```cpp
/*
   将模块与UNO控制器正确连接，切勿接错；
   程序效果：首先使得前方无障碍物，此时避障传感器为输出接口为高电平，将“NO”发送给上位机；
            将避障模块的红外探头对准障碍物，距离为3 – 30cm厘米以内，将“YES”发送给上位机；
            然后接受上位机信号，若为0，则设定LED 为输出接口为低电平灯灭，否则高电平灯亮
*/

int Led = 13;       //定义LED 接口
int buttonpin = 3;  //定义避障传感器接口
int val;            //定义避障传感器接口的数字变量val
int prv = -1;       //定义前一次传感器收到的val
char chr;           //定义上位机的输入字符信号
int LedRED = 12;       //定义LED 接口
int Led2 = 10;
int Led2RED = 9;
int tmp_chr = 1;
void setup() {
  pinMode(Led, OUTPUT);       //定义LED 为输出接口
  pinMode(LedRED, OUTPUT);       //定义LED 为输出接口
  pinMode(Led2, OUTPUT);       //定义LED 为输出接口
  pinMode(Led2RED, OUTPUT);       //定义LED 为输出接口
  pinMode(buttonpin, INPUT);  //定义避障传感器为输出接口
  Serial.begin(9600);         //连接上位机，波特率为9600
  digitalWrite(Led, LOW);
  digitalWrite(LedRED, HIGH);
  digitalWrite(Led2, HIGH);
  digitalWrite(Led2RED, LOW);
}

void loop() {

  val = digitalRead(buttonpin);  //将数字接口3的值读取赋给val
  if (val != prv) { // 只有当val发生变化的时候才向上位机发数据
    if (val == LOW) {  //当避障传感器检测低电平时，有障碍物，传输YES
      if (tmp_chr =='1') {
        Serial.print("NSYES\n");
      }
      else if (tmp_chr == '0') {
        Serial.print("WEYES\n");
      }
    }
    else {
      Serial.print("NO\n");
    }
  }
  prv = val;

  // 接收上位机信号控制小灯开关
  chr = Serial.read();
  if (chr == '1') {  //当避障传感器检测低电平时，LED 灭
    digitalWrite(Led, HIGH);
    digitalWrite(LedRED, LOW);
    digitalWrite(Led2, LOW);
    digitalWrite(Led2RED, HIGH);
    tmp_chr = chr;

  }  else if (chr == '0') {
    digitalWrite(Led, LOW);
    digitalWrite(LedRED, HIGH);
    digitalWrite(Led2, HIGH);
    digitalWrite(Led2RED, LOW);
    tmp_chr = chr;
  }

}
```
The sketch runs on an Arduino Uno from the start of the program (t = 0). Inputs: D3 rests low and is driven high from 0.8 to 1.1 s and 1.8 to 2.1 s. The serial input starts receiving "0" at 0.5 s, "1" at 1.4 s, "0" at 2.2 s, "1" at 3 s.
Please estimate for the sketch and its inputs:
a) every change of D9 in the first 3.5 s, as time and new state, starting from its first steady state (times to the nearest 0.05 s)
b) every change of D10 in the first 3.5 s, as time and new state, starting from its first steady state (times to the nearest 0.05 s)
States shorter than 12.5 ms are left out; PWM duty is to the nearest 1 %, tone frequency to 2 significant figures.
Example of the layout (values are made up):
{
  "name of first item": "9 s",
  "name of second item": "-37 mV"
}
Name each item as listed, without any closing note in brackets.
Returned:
{
  "every change of D9 in the first 3.5 s, as time and new state, starting from its first steady state": "0 s low; 1.4 s high; 2.2 s low; 3 s high",
  "every change of D10 in the first 3.5 s, as time and new state, starting from its first steady state": "0 s high; 1.4 s low; 2.2 s high; 3 s low"
}
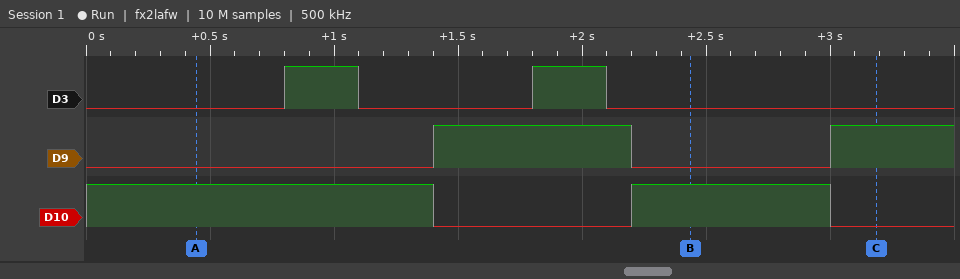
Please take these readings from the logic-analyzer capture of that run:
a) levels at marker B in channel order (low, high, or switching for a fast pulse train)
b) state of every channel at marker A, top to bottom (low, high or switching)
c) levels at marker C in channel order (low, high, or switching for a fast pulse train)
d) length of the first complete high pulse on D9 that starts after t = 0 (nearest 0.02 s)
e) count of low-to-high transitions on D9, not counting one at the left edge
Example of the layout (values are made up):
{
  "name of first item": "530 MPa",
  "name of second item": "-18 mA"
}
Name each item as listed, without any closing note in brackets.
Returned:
{
  "levels at marker B in channel order": "D3 low, D9 low, D10 high",
  "state of every channel at marker A, top to bottom": "D3 low, D9 low, D10 high",
  "levels at marker C in channel order": "D3 low, D9 high, D10 low",
  "length of the first complete high pulse on D9 that starts after t = 0": "0.80 s",
  "count of low-to-high transitions on D9, not counting one at the left edge": "2"
}
